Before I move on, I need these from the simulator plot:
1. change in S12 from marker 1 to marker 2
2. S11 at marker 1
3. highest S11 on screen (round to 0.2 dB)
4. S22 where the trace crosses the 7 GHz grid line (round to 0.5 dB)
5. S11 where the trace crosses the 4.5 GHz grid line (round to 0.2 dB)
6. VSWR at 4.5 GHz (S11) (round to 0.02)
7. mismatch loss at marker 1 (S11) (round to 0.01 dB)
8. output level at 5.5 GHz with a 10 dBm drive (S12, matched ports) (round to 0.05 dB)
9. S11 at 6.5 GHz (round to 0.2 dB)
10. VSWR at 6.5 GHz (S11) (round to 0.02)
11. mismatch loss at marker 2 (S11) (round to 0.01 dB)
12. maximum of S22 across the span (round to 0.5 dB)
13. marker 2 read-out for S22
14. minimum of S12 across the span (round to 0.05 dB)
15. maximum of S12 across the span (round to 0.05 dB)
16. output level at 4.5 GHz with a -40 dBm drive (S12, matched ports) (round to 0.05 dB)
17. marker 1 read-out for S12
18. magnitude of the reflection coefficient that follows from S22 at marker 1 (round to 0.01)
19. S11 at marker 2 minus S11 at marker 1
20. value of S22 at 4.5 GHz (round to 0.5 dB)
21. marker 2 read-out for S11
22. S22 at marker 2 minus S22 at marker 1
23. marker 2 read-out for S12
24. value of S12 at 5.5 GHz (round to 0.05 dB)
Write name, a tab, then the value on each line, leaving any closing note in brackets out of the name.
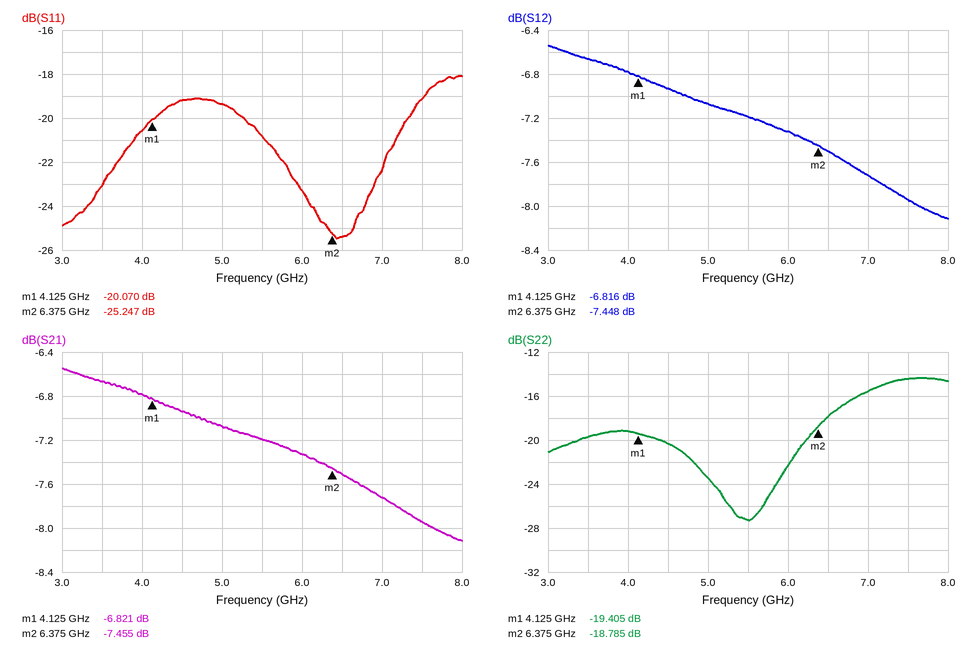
change in S12 from marker 1 to marker 2	-0.632 dB
S11 at marker 1	-20.070 dB
highest S11 on screen	-18.0 dB
S22 where the trace crosses the 7 GHz grid line	-15.5 dB
S11 where the trace crosses the 4.5 GHz grid line	-19.2 dB
VSWR at 4.5 GHz (S11)	1.24
mismatch loss at marker 1 (S11)	0.04 dB
output level at 5.5 GHz with a 10 dBm drive (S12, matched ports)	2.80 dBm
S11 at 6.5 GHz	-25.4 dB
VSWR at 6.5 GHz (S11)	1.12
mismatch loss at marker 2 (S11)	0.01 dB
maximum of S22 across the span	-14.5 dB
marker 2 read-out for S22	-18.785 dB
minimum of S12 across the span	-8.10 dB
maximum of S12 across the span	-6.55 dB
output level at 4.5 GHz with a -40 dBm drive (S12, matched ports)	-46.95 dBm
marker 1 read-out for S12	-6.816 dB
magnitude of the reflection coefficient that follows from S22 at marker 1	0.11
S11 at marker 2 minus S11 at marker 1	-5.177 dB
value of S22 at 4.5 GHz	-20.5 dB
marker 2 read-out for S11	-25.247 dB
S22 at marker 2 minus S22 at marker 1	0.620 dB
marker 2 read-out for S12	-7.448 dB
value of S12 at 5.5 GHz	-7.20 dB
